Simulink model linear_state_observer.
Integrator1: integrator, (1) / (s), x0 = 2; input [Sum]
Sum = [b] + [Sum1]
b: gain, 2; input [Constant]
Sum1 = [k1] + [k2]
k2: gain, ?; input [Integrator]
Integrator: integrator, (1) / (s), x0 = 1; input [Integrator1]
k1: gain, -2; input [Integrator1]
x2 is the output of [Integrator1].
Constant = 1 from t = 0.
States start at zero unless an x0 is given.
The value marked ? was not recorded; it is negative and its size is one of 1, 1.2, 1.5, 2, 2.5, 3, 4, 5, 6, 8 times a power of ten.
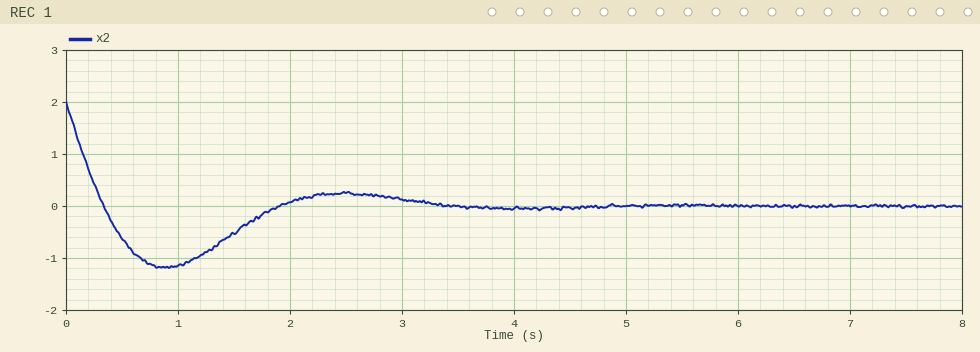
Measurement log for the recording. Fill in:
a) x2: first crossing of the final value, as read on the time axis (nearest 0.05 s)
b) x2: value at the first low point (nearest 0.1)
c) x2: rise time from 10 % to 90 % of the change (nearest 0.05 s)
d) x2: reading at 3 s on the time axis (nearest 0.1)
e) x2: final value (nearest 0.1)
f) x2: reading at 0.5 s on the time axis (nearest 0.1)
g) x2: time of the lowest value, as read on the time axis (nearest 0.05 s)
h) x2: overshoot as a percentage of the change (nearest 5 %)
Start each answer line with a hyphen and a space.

- 0.35 s
- -1.2
- 0.25 s
- 0.1
- 0.0
- -0.6
- 0.90 s
- 60 %
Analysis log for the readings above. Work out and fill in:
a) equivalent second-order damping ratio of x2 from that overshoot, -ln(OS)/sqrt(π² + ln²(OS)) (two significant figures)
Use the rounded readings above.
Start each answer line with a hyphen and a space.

- 0.16
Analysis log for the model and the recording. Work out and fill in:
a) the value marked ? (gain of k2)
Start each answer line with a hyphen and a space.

- -5
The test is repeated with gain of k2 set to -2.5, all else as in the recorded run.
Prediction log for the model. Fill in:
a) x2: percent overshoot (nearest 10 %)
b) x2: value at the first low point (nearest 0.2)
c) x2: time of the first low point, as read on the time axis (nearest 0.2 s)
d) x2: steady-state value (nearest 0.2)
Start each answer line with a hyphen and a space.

- 30 %
- -0.6
- 1.4 s
- 0.0
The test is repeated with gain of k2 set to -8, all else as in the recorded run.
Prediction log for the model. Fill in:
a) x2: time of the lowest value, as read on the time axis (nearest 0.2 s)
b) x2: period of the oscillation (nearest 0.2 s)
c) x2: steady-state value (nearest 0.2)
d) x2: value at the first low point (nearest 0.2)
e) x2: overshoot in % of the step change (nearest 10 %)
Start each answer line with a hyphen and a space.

- 0.6 s
- 2.4 s
- 0.0
- -1.8
- 90 %
